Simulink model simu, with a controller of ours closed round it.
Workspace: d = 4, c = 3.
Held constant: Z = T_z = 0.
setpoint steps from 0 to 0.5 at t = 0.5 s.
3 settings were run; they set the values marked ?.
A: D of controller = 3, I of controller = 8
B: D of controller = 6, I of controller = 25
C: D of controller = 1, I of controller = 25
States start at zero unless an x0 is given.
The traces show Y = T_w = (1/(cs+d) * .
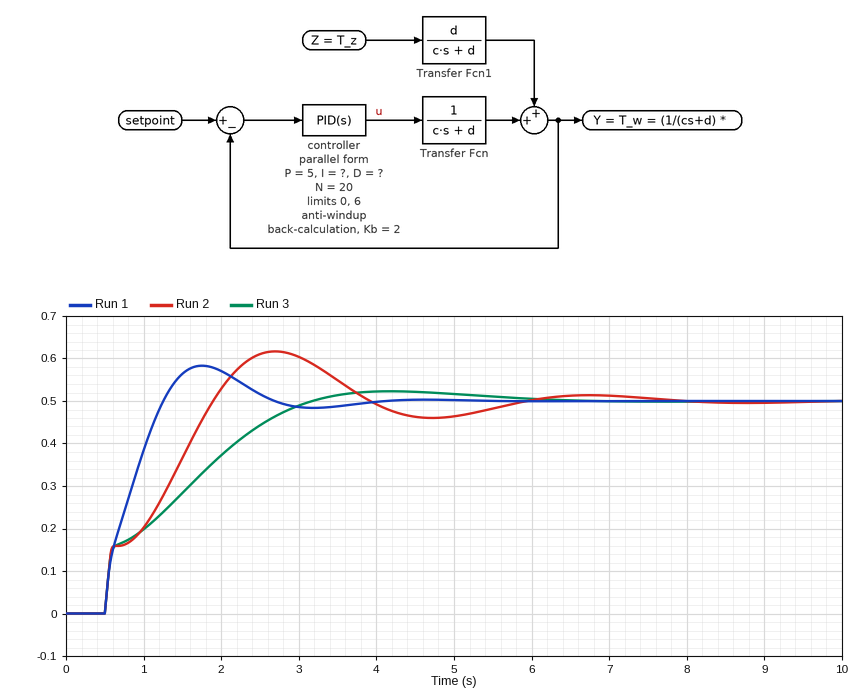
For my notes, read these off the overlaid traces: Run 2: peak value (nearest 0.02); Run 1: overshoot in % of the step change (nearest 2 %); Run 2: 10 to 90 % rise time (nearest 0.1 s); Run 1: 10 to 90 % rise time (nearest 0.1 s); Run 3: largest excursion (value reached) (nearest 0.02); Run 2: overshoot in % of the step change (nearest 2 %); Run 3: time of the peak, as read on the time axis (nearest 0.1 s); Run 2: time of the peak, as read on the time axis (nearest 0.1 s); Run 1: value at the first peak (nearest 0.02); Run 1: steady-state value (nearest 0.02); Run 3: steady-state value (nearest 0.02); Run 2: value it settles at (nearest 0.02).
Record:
0.62
16 %
1.2 s
0.6 s
0.52
24 %
4.2 s
2.7 s
0.58
0.50
0.50
0.50
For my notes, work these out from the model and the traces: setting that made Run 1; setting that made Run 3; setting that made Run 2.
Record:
C
A
B
